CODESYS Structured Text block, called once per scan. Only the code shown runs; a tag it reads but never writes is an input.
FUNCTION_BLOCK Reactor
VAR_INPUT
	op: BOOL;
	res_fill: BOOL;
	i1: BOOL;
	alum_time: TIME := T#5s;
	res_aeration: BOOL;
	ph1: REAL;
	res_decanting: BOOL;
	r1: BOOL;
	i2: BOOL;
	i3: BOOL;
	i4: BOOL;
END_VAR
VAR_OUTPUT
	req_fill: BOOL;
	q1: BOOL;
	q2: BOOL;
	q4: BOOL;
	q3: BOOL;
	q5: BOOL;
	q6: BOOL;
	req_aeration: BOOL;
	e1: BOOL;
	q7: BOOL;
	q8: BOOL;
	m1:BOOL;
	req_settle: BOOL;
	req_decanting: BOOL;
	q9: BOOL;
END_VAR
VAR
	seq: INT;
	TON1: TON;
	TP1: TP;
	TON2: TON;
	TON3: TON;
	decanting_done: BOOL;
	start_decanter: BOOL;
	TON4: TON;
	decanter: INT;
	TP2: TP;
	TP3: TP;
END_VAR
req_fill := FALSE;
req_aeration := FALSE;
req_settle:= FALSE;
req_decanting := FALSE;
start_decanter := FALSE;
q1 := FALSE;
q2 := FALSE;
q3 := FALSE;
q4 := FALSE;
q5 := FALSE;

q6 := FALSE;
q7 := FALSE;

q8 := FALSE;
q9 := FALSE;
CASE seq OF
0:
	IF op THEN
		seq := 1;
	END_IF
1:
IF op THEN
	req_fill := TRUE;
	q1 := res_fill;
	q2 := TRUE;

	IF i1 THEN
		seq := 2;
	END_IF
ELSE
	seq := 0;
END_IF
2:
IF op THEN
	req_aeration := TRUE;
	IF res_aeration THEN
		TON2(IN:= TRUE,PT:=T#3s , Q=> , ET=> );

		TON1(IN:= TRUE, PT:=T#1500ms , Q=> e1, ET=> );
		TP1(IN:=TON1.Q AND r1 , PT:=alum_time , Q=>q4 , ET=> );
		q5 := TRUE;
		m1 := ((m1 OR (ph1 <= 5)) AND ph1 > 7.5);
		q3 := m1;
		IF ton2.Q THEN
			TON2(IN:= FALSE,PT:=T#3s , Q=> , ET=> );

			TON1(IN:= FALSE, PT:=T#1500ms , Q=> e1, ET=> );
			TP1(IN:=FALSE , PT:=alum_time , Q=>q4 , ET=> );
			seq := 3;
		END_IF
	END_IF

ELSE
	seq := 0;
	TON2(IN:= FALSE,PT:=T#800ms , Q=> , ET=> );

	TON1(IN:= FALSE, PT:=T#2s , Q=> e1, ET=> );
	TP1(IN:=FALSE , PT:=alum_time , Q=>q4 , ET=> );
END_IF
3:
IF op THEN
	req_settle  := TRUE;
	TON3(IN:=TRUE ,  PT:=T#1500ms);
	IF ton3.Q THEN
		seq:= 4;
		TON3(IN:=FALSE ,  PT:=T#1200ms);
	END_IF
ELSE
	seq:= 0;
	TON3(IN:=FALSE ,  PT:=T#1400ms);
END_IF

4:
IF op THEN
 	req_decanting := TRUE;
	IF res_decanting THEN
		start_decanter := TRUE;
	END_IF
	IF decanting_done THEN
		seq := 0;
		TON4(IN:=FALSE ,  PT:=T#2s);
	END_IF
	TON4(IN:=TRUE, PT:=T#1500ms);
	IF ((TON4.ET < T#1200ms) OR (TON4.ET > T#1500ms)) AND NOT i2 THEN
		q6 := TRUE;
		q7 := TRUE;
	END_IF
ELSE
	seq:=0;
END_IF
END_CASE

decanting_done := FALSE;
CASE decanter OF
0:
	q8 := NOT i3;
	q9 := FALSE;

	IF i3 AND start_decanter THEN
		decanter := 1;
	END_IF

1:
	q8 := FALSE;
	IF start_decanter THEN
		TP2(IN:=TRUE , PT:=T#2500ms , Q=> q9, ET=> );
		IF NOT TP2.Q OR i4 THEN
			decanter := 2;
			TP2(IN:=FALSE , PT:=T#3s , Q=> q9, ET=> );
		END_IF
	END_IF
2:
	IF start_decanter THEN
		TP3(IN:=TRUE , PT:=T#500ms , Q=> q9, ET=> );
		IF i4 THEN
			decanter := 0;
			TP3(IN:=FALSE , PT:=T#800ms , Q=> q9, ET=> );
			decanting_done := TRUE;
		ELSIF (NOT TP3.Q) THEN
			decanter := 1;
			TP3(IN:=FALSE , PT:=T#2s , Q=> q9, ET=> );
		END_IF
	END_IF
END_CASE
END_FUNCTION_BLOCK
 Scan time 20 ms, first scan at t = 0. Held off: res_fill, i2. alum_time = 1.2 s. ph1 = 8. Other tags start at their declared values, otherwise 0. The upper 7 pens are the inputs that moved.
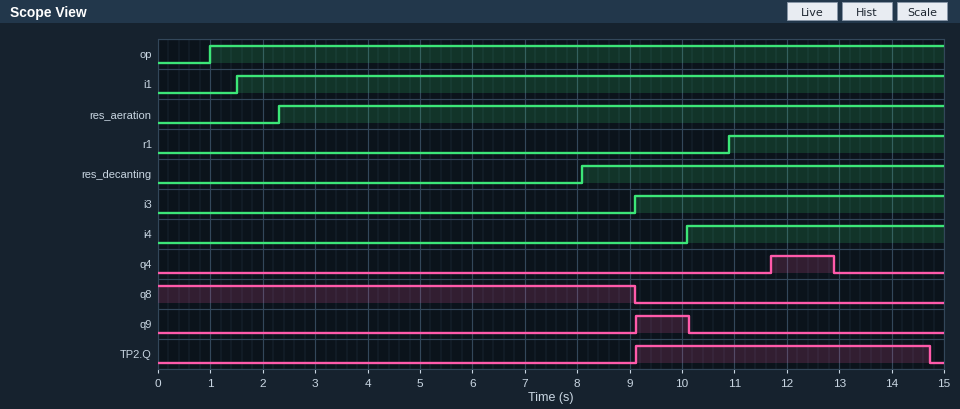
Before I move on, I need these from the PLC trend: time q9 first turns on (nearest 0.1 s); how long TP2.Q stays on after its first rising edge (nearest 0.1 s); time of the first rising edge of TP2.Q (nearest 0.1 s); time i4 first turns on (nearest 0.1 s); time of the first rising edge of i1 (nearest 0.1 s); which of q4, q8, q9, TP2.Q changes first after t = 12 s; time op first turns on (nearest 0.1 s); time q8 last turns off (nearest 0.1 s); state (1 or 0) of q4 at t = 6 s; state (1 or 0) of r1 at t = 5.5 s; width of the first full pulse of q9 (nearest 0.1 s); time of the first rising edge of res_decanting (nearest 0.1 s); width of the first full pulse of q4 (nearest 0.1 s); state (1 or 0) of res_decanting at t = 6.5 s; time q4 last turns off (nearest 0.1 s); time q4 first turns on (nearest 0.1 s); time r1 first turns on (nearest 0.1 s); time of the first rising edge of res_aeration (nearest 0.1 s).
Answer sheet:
9.1 s
5.6 s
9.1 s
10.1 s
1.5 s
q4
1.0 s
9.1 s
0
0
1.0 s
8.1 s
1.2 s
0
12.9 s
11.7 s
10.9 s
2.3 s
